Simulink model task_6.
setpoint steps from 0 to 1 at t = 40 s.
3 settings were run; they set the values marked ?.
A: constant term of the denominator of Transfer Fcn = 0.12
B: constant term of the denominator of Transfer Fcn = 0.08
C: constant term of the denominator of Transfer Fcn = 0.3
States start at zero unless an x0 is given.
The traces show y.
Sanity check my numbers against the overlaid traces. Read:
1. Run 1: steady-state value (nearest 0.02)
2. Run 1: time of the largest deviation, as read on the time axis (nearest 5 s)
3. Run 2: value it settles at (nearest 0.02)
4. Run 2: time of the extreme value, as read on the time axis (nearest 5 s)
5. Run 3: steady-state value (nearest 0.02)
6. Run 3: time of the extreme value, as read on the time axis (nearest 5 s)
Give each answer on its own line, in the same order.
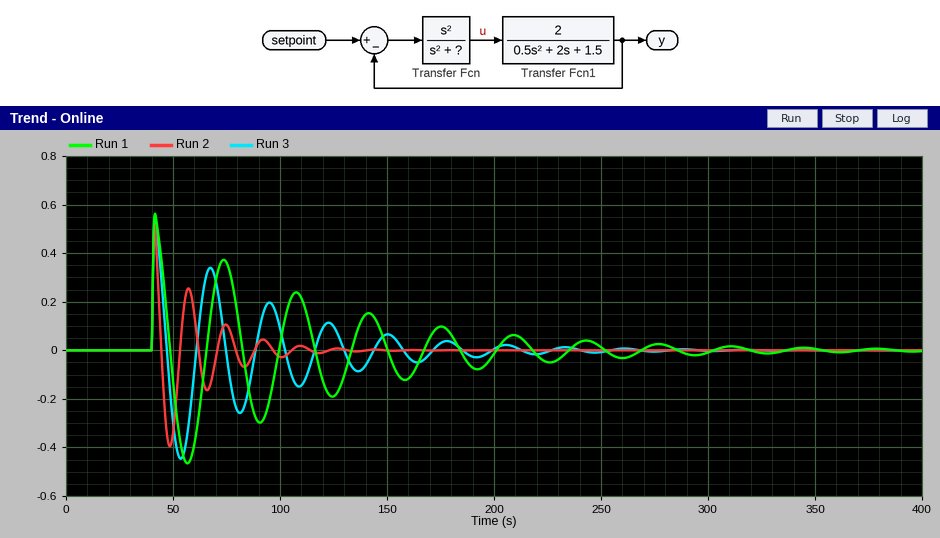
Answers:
0.00
40 s
0.00
40 s
0.00
40 s
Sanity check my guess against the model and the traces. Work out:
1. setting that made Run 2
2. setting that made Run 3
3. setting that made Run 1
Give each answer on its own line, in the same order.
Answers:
C
A
B
